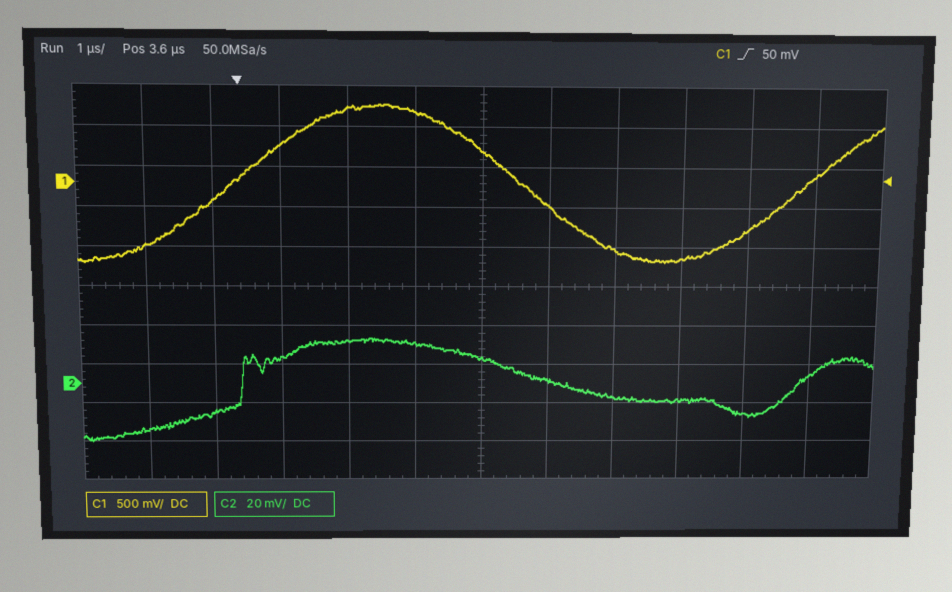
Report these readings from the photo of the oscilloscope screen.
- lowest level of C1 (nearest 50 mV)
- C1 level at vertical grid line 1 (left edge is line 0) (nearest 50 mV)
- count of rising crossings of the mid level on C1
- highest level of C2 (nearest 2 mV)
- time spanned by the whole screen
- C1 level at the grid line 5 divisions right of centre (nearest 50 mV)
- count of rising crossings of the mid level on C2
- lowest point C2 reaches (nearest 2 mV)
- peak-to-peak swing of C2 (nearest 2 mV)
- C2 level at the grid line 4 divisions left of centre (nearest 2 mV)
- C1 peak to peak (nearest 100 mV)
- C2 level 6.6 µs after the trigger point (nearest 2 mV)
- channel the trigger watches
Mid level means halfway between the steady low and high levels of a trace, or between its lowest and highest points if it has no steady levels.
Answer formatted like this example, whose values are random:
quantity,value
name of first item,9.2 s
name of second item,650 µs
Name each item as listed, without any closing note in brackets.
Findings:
quantity,value
lowest level of C1,-1.00 V
C1 level at vertical grid line 1 (left edge is line 0),-800 mV
count of rising crossings of the mid level on C1,2
highest level of C2,24 mV
time spanned by the whole screen,12 µs
C1 level at the grid line 5 divisions right of centre,100 mV
count of rising crossings of the mid level on C2,2
lowest point C2 reaches,-30 mV
peak-to-peak swing of C2,54 mV
C2 level at the grid line 4 divisions left of centre,-14 mV
C1 peak to peak,2.00 V
C2 level 6.6 µs after the trigger point,-8 mV
channel the trigger watches,C1
